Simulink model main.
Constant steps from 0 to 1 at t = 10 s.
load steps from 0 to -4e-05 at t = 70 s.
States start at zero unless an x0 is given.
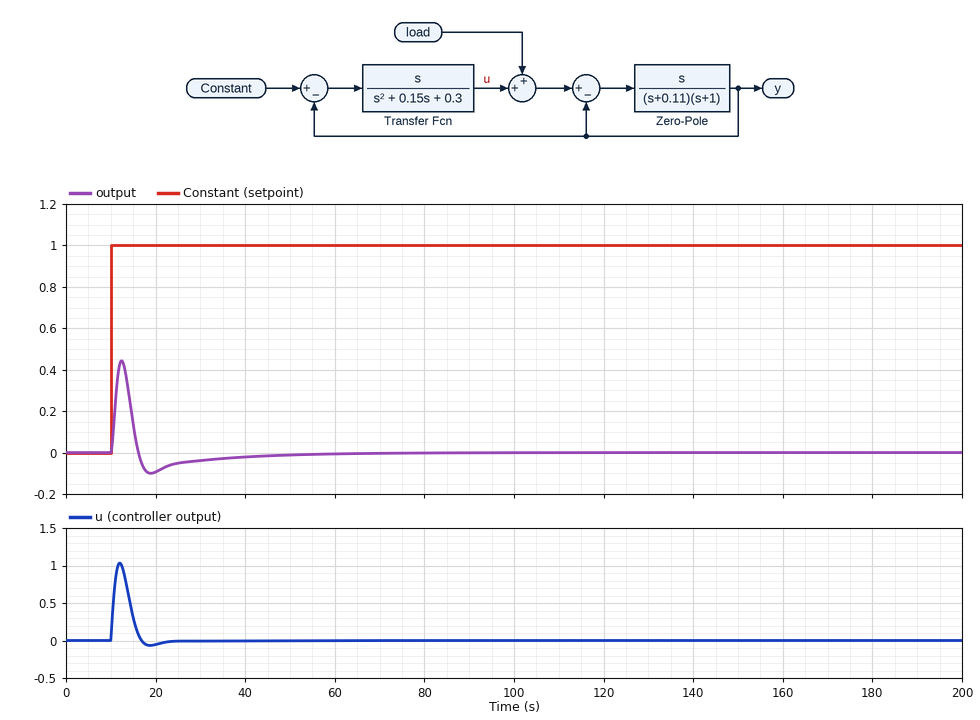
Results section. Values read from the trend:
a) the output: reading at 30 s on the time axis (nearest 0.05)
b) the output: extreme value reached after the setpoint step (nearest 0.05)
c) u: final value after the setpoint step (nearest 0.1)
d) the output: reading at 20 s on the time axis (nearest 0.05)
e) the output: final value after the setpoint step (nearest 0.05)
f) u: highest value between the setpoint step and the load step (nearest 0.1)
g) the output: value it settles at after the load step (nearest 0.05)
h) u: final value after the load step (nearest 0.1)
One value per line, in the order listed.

-0.05
0.45
0.0
-0.10
0.00
1.0
0.00
0.0
